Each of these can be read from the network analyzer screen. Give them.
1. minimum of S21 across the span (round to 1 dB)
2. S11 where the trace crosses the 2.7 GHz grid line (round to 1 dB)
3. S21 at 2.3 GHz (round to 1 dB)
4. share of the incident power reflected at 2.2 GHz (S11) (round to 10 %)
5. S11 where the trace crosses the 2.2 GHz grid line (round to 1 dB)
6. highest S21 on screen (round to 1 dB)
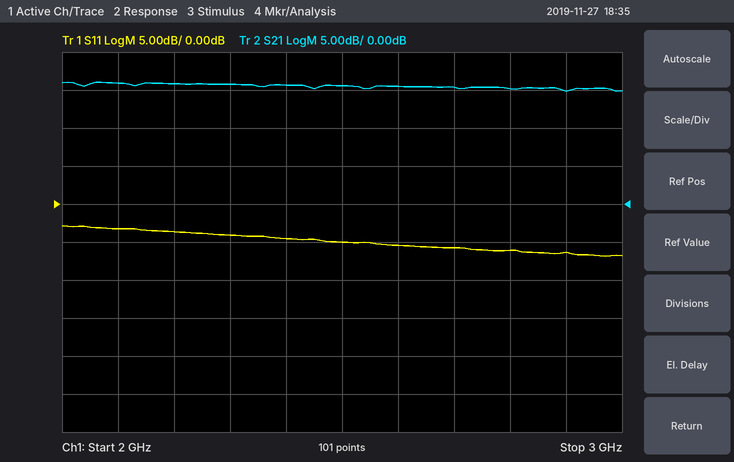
15 dB
-6 dB
16 dB
40 %
-4 dB
16 dB
